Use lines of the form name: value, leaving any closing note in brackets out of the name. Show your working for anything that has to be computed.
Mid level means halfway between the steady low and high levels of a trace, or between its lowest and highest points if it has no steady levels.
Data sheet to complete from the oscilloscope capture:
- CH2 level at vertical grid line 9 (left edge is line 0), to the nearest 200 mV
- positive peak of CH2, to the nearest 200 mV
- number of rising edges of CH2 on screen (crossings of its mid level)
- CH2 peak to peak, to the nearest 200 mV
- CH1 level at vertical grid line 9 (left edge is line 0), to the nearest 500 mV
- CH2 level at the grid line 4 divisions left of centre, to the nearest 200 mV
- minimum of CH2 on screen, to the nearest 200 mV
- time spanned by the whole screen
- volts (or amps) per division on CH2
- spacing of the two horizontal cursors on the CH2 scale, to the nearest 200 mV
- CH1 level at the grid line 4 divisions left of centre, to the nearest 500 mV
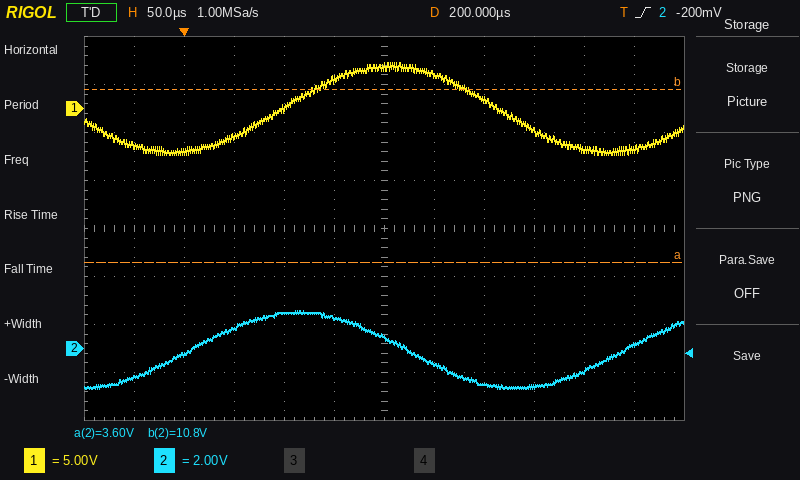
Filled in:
CH2 level at vertical grid line 9 (left edge is line 0), to the nearest 200 mV: -1.6 V
positive peak of CH2, to the nearest 200 mV: 1.6 V
number of rising edges of CH2 on screen: 2
CH2 peak to peak, to the nearest 200 mV: 1.6 V − (-1.6 V) = 3.2 V
CH1 level at vertical grid line 9 (left edge is line 0), to the nearest 500 mV: -2.5 V
CH2 level at the grid line 4 divisions left of centre, to the nearest 200 mV: -200 mV
minimum of CH2 on screen, to the nearest 200 mV: -1.6 V
time spanned by the whole screen: 600 µs
volts (or amps) per division on CH2: 2 V
spacing of the two horizontal cursors on the CH2 scale, to the nearest 200 mV: 7.2 V
CH1 level at the grid line 4 divisions left of centre, to the nearest 500 mV: -4.5 V
